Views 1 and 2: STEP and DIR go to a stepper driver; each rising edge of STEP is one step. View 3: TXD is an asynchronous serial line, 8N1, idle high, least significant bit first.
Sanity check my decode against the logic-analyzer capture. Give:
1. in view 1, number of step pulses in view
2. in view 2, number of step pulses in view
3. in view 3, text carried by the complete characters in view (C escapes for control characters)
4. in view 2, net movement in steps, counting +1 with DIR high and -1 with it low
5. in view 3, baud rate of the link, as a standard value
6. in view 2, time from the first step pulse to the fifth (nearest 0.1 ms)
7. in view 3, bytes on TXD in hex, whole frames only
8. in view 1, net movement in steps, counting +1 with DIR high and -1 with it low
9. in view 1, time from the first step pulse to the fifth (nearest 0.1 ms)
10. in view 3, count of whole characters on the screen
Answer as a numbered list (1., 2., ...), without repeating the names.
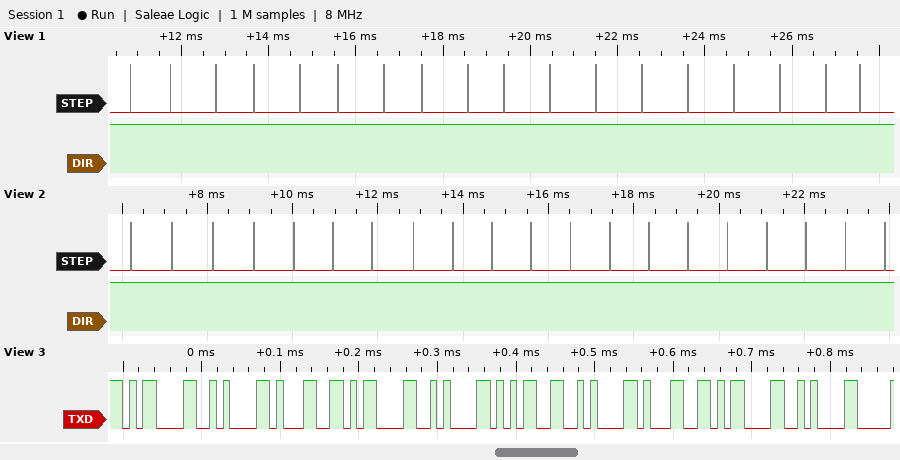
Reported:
1. 18
2. 20
3. "\r\n1\r\n5\n1\r\n"
4. +20
5. 115200 baud
6. 3.8 ms
7. 0D 0A 31 0D 0A 35 0A 31 0D 0A
8. +18
9. 3.9 ms
10. 10
